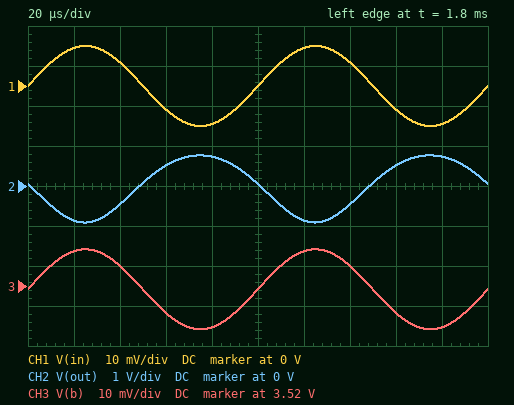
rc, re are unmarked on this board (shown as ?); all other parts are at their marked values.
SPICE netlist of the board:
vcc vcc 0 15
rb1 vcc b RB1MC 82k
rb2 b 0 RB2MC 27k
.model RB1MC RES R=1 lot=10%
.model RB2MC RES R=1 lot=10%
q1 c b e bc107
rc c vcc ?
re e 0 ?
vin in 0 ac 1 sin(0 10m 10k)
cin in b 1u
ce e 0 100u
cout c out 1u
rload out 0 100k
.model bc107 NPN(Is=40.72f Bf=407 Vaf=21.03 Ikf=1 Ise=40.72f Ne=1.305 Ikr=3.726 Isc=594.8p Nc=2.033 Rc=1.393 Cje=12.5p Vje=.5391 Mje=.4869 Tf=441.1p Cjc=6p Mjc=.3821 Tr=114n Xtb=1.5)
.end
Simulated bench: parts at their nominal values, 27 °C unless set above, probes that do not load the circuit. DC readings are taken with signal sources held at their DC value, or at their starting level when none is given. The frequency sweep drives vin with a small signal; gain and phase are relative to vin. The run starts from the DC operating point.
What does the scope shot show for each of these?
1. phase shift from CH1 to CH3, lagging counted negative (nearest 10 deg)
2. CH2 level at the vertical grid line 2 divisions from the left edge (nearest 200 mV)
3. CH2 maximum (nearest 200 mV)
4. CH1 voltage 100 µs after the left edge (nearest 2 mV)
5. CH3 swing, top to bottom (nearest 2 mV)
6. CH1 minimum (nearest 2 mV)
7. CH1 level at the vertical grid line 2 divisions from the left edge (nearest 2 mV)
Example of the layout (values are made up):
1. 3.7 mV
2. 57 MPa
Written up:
1. 0 deg
2. -400 mV
3. 800 mV
4. 0 V
5. 20 mV
6. -10 mV
7. 6 mV
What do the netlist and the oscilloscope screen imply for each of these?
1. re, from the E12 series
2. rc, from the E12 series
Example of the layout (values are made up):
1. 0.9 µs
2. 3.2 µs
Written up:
1. 1.2 kΩ
2. 1 kΩ
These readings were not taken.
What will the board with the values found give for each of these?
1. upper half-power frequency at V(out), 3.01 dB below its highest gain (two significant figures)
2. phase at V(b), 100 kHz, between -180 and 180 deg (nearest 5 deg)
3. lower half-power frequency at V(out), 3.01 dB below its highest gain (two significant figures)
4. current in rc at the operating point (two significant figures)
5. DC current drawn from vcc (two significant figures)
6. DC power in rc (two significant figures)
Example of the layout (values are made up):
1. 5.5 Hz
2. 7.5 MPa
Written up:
1. 77 MHz
2. 0 deg
3. 190 Hz
4. 2.4 mA
5. 2.5 mA
6. 5.7 mW
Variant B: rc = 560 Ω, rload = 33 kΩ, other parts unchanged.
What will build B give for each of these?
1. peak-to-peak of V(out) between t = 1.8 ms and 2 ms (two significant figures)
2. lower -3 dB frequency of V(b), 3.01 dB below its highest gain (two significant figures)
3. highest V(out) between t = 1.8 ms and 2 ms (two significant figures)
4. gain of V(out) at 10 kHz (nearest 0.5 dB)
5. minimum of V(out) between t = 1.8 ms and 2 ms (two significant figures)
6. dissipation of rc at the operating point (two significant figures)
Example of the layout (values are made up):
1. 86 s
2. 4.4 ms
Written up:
1. 970 mV
2. 20 Hz
3. 440 mV
4. 34.0 dB
5. -530 mV
6. 3.2 mW
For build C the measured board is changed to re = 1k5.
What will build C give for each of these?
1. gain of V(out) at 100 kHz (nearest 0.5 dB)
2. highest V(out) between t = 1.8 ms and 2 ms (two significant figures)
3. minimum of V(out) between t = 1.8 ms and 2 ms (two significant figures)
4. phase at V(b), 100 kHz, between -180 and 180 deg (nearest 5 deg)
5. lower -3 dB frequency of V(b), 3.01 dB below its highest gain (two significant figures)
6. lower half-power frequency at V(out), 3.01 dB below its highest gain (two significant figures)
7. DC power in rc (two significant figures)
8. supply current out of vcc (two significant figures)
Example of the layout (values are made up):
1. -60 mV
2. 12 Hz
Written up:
1. 37.0 dB
2. 630 mV
3. -760 mV
4. 0 deg
5. 24 Hz
6. 160 Hz
7. 3.8 mW
8. 2.1 mA
